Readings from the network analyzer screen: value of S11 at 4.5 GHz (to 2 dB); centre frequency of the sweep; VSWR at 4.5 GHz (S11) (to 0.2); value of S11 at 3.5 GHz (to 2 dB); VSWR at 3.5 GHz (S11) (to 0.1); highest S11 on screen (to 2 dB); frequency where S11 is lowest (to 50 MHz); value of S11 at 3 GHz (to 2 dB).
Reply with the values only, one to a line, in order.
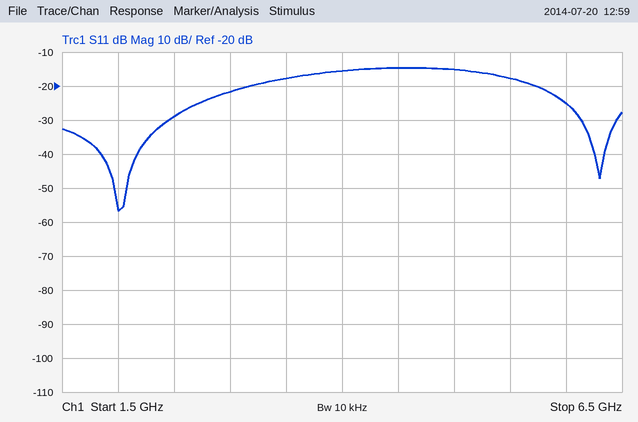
-14 dB
4 GHz
1.4
-18 dB
1.3
-14 dB
2.00 GHz
-22 dB
